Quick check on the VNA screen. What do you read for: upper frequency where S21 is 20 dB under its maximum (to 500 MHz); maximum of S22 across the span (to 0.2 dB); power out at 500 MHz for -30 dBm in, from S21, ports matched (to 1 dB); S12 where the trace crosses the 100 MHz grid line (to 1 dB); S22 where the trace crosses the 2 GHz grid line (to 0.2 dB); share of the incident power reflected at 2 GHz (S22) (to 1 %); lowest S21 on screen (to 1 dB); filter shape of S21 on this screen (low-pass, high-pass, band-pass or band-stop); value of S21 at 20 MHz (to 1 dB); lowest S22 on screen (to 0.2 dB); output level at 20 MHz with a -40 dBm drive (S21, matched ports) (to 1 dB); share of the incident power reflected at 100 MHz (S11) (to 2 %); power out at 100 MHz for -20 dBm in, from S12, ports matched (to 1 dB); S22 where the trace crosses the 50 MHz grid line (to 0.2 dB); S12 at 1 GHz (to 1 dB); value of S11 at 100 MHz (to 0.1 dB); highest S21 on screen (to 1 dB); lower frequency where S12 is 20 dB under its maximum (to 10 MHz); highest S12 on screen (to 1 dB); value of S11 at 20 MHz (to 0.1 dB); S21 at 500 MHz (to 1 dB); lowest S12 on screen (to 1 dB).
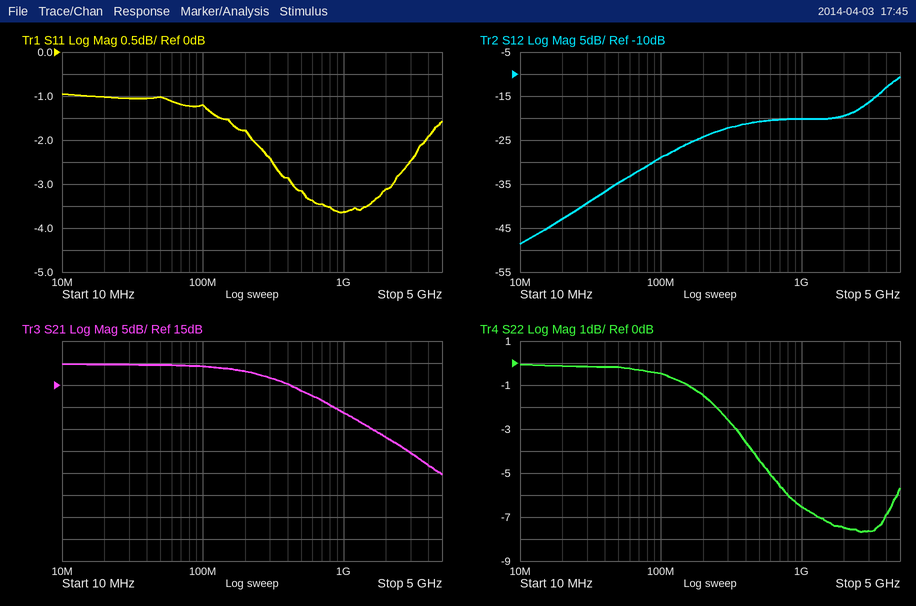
3.0 GHz
0.0 dB
-16 dBm
-29 dB
-7.4 dB
18 %
-5 dB
low-pass
20 dB
-7.6 dB
-20 dBm
76 %
-49 dBm
-0.2 dB
-20 dB
-1.2 dB
20 dB
80 MHz
-11 dB
-1.0 dB
14 dB
-49 dB
